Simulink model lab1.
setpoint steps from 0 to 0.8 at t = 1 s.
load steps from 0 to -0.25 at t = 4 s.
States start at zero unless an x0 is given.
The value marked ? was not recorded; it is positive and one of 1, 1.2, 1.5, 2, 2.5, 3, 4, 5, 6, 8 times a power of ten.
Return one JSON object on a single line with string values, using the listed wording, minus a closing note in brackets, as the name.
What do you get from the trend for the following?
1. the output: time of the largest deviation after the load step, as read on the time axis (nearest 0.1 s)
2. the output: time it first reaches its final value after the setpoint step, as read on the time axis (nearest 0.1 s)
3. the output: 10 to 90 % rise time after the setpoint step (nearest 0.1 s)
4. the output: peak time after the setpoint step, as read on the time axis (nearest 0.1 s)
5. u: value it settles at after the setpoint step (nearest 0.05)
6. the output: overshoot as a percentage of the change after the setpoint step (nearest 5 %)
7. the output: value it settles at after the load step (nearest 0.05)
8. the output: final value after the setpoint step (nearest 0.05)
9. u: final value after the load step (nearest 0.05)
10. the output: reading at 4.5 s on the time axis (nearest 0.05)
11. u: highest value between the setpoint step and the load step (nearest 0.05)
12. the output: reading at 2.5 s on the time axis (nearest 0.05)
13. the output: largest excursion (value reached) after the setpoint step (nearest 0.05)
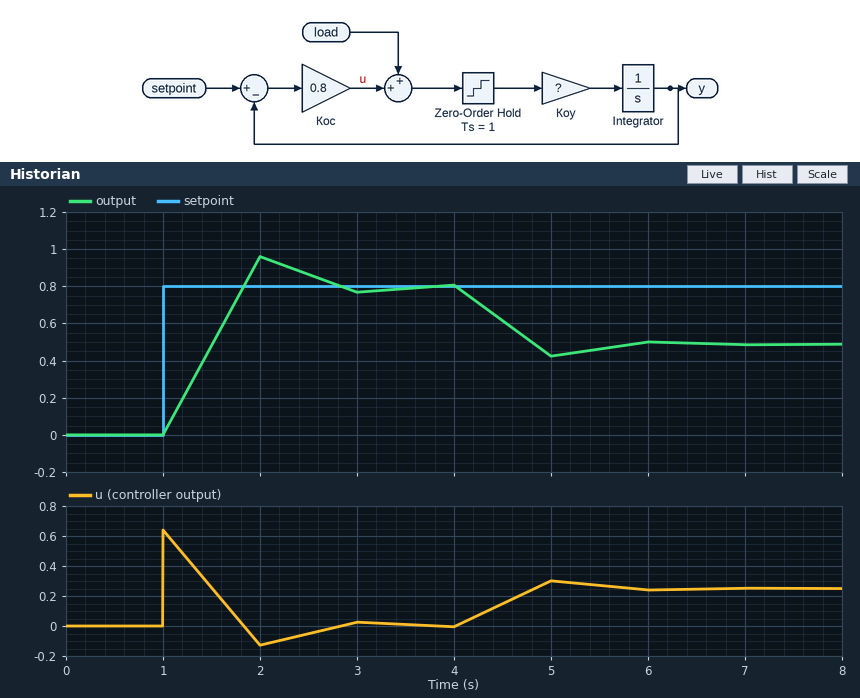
{"the output: time of the largest deviation after the load step, as read on the time axis": "5.0 s", "the output: time it first reaches its final value after the setpoint step, as read on the time axis": "1.8 s", "the output: 10 to 90 % rise time after the setpoint step": "0.7 s", "the output: peak time after the setpoint step, as read on the time axis": "2.0 s", "u: value it settles at after the setpoint step": "0.00", "the output: overshoot as a percentage of the change after the setpoint step": "20 %", "the output: value it settles at after the load step": "0.50", "the output: final value after the setpoint step": "0.80", "u: final value after the load step": "0.25", "the output: reading at 4.5 s on the time axis": "0.60", "u: highest value between the setpoint step and the load step": "0.65", "the output: reading at 2.5 s on the time axis": "0.85", "the output: largest excursion (value reached) after the setpoint step": "0.95"}
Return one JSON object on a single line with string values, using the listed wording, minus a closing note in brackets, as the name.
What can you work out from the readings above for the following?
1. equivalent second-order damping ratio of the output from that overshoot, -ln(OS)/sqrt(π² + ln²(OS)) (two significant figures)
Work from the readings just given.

{"equivalent second-order damping ratio of the output from that overshoot, -ln(OS)/sqrt(π² + ln²(OS))": "0.46"}
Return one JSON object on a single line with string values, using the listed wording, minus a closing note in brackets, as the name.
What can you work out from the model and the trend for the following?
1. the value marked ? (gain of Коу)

{"the value marked ?": "1.5"}
